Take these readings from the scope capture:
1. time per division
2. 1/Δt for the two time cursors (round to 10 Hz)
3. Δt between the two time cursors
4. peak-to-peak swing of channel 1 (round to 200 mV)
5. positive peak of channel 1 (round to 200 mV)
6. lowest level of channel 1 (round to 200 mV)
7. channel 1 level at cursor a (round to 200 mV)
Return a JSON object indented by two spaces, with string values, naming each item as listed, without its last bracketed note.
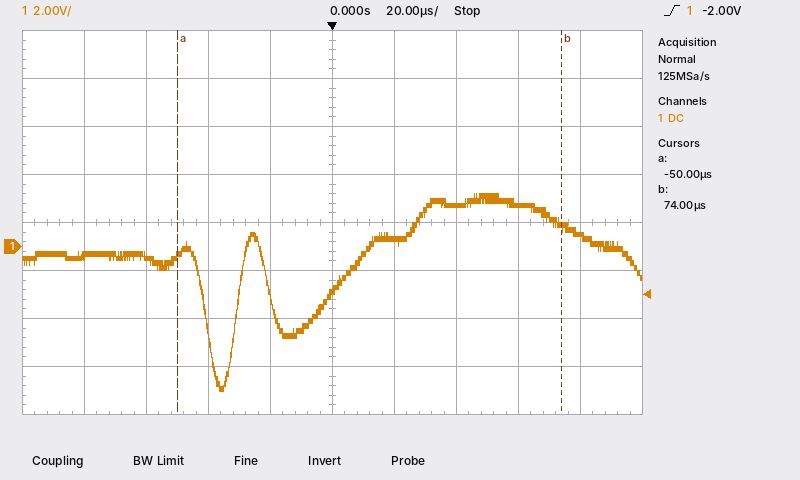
{
  "time per division": "20 µs",
  "1/Δt for the two time cursors": "8.06 kHz",
  "Δt between the two time cursors": "124 µs",
  "peak-to-peak swing of channel 1": "8.2 V",
  "positive peak of channel 1": "2.2 V",
  "lowest level of channel 1": "-6.0 V",
  "channel 1 level at cursor a": "-400 mV"
}
